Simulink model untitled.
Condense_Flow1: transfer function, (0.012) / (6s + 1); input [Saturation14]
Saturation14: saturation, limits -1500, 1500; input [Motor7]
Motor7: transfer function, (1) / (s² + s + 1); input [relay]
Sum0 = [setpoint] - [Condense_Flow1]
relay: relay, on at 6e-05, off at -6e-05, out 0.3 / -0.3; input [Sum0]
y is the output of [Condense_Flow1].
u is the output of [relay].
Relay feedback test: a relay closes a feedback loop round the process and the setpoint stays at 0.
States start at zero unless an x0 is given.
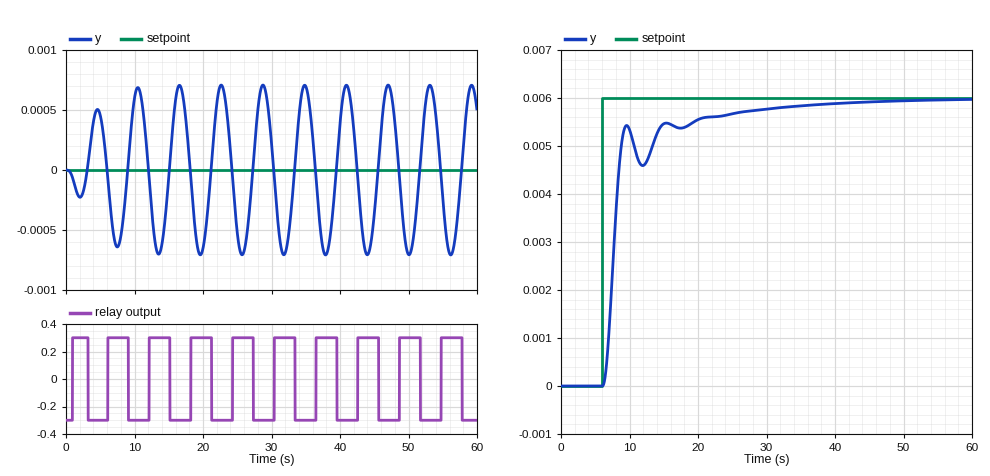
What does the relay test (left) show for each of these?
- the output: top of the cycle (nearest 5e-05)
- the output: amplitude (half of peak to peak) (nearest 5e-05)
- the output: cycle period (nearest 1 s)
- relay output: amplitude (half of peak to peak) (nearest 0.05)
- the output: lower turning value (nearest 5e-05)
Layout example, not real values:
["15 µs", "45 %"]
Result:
["0.00070", "0.00070", "6 s", "0.30", "-0.00070"]
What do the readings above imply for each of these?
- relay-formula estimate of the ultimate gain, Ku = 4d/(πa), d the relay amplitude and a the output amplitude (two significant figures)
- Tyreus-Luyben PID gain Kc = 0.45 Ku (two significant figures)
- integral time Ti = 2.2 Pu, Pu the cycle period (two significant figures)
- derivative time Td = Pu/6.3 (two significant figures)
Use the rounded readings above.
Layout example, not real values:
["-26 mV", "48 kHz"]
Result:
["550", "250", "13 s", "0.95 s"]
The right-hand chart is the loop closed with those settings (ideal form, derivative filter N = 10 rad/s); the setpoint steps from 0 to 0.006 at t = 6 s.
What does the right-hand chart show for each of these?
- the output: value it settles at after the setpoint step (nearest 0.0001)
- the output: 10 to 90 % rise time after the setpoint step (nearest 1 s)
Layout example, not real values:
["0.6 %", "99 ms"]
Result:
["0.0060", "3 s"]
